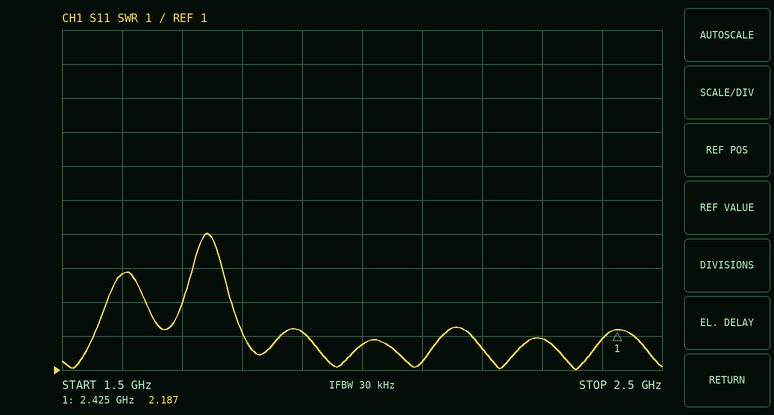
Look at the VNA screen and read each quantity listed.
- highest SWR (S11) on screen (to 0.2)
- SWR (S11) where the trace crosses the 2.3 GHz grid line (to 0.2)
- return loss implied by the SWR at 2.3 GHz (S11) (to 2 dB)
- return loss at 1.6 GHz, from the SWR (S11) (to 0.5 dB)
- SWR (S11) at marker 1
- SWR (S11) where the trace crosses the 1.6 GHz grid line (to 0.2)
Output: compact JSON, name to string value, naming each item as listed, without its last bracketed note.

{"highest SWR (S11) on screen": "5.0", "SWR (S11) where the trace crosses the 2.3 GHz grid line": "2.0", "return loss implied by the SWR at 2.3 GHz (S11)": "10 dB", "return loss at 1.6 GHz, from the SWR (S11)": "4.5 dB", "SWR (S11) at marker 1": "2.187", "SWR (S11) where the trace crosses the 1.6 GHz grid line": "3.8"}
